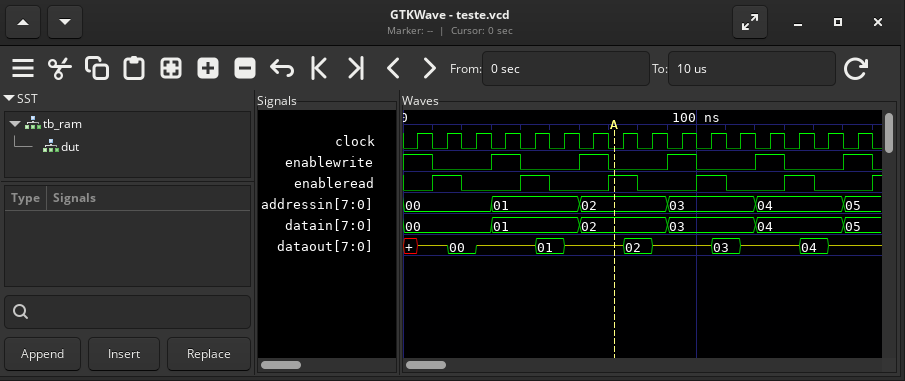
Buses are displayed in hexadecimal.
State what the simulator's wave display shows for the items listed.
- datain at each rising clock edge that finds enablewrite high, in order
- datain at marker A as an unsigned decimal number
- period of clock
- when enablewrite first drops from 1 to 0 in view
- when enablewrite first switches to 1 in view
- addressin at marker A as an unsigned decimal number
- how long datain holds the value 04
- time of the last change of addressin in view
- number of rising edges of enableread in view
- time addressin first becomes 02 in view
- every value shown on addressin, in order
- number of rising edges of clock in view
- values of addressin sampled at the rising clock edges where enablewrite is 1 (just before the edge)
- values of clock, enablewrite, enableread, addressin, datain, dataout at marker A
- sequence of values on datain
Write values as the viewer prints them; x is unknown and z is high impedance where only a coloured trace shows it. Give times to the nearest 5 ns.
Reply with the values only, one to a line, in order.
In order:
00, 01, 02, 03, 04, 05
2
10 ns
10 ns
30 ns
2
30 ns
150 ns
6
60 ns
00, 01, 02, 03, 04, 05
16
00, 01, 02, 03, 04, 05
clock=0, enablewrite=0, enableread=1, addressin=02, datain=02, dataout=z
00, 01, 02, 03, 04, 05
